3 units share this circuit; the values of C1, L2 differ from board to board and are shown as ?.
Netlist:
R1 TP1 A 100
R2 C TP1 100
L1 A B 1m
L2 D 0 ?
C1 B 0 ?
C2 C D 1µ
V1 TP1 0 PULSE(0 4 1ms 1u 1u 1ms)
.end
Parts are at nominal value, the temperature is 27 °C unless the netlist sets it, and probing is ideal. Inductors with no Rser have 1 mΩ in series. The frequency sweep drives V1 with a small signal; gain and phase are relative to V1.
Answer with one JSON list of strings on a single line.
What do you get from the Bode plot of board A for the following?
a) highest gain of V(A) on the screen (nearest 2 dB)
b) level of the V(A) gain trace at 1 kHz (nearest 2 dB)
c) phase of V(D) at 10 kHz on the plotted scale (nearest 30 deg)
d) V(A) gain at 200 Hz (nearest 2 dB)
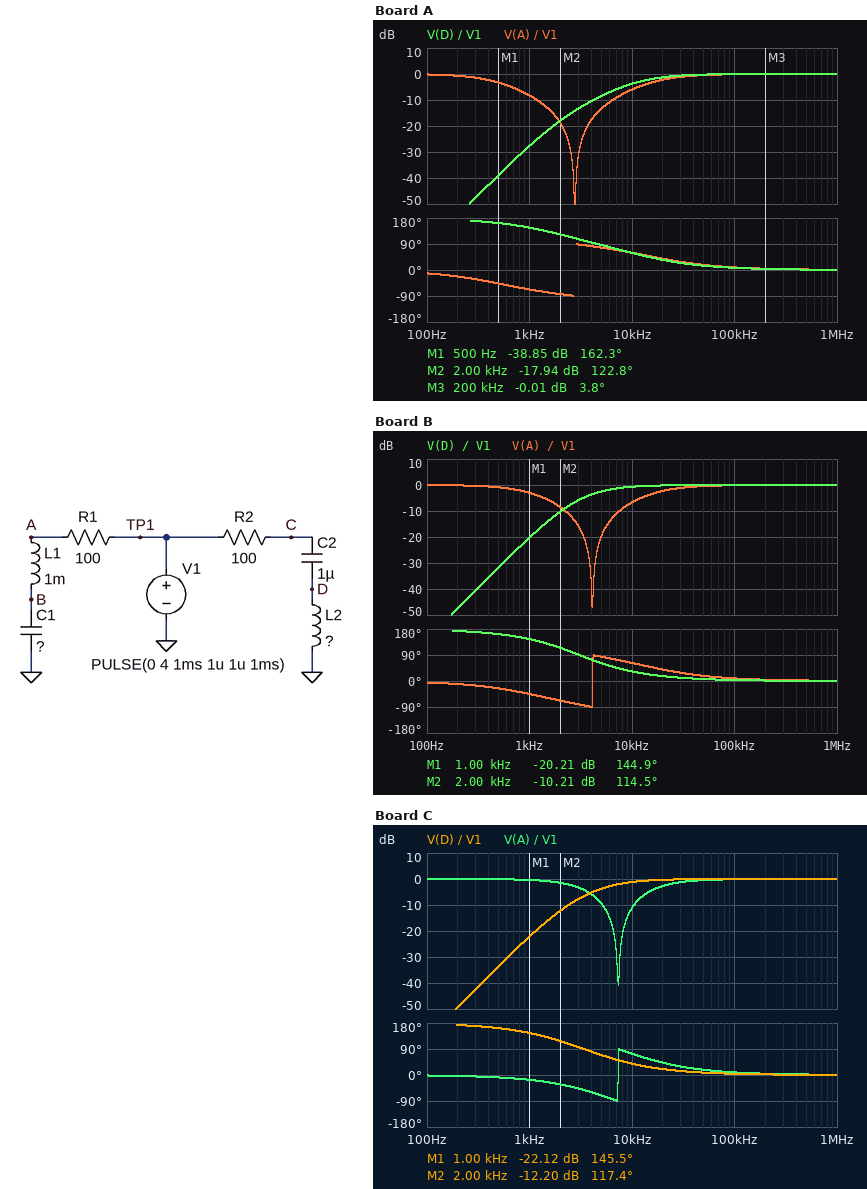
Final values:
["0 dB", "-8 dB", "60 deg", "0 dB"]
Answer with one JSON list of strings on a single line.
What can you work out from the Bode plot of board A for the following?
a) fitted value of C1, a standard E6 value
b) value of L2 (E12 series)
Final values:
["3.3 µF", "1.2 mH"]
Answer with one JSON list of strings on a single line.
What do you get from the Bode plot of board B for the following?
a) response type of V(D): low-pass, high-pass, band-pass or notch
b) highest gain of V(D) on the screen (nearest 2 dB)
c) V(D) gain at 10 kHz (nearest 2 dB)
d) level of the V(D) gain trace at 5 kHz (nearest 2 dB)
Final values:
["high-pass", "0 dB", "0 dB", "-2 dB"]
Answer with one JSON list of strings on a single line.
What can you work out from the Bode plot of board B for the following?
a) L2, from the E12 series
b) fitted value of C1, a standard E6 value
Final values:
["2.7 mH", "1.5 µF"]
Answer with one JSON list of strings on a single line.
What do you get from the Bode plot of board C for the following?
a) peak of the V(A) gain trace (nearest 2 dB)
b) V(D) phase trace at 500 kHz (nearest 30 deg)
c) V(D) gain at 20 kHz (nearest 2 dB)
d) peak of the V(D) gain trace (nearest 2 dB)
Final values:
["0 dB", "0 deg", "0 dB", "0 dB"]
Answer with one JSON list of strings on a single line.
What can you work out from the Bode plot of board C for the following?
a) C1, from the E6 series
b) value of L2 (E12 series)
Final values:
["470 nF", "2.2 mH"]
